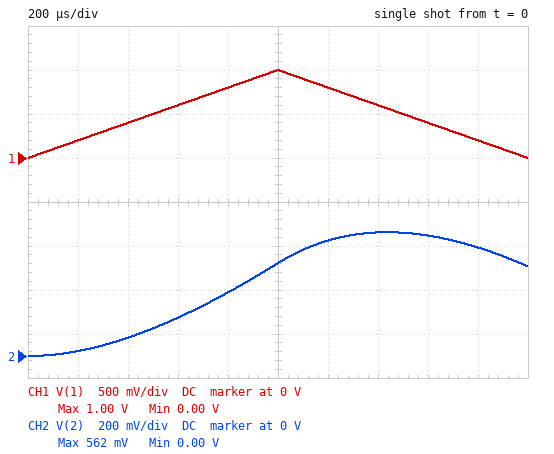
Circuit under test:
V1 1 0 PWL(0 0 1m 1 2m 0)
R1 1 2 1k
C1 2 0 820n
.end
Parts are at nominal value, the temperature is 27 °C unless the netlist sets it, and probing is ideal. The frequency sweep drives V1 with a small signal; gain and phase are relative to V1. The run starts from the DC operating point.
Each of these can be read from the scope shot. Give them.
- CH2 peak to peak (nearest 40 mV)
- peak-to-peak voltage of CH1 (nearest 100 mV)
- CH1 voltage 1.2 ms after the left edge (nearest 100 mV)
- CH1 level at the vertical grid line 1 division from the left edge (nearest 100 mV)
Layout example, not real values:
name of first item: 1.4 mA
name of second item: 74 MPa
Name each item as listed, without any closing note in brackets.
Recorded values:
CH2 peak to peak: 560 mV
peak-to-peak voltage of CH1: 1.0 V
CH1 voltage 1.2 ms after the left edge: 800 mV
CH1 level at the vertical grid line 1 division from the left edge: 200 mV
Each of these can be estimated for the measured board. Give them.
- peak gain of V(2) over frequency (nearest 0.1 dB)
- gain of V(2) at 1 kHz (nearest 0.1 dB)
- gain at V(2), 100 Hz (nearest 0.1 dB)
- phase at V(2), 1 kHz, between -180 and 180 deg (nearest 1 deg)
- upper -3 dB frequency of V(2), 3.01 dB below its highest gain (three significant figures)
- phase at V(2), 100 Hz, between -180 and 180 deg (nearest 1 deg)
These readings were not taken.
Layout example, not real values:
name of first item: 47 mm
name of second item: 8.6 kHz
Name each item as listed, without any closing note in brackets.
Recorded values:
peak gain of V(2) over frequency: 0 dB
gain of V(2) at 1 kHz: -14.4 dB
gain at V(2), 100 Hz: -1.0 dB
phase at V(2), 1 kHz, between -180 and 180 deg: -79 deg
upper -3 dB frequency of V(2), 3.01 dB below its highest gain: 194 Hz
phase at V(2), 100 Hz, between -180 and 180 deg: -27 deg
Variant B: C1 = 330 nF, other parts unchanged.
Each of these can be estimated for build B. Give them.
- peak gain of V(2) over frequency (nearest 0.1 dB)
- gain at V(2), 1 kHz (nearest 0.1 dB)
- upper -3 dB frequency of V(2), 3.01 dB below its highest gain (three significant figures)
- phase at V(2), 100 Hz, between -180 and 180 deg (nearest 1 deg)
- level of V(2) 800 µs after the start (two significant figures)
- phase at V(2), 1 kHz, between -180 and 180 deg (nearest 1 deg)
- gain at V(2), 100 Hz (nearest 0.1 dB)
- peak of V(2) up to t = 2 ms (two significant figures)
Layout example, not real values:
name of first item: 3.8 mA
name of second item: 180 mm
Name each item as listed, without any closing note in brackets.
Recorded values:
peak gain of V(2) over frequency: 0 dB
gain at V(2), 1 kHz: -7.2 dB
upper -3 dB frequency of V(2), 3.01 dB below its highest gain: 482 Hz
phase at V(2), 100 Hz, between -180 and 180 deg: -12 deg
level of V(2) 800 µs after the start: 500 mV
phase at V(2), 1 kHz, between -180 and 180 deg: -64 deg
gain at V(2), 100 Hz: -0.2 dB
peak of V(2) up to t = 2 ms: 780 mV
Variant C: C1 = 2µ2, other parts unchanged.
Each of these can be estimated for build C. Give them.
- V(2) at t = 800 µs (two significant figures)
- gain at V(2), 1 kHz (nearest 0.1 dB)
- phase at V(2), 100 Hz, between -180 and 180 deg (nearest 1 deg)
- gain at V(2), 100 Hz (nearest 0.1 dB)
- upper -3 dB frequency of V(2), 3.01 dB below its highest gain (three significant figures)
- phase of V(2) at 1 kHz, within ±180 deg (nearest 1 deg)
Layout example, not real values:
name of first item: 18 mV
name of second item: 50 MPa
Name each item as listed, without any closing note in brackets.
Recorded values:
V(2) at t = 800 µs: 130 mV
gain at V(2), 1 kHz: -22.8 dB
phase at V(2), 100 Hz, between -180 and 180 deg: -54 deg
gain at V(2), 100 Hz: -4.6 dB
upper -3 dB frequency of V(2), 3.01 dB below its highest gain: 72.3 Hz
phase of V(2) at 1 kHz, within ±180 deg: -86 deg
